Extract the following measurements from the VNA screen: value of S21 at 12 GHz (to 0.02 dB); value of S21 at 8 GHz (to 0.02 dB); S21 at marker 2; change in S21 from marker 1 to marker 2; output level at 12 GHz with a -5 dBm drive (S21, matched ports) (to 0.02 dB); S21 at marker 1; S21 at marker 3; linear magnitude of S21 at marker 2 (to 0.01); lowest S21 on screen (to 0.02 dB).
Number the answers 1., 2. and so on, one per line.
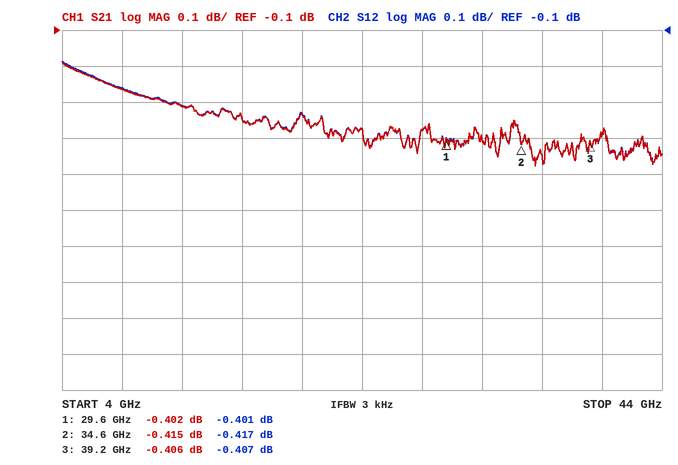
1. -0.32 dB
2. -0.26 dB
3. -0.415 dB
4. -0.013 dB
5. -5.32 dBm
6. -0.402 dB
7. -0.406 dB
8. 0.95
9. -0.48 dB
